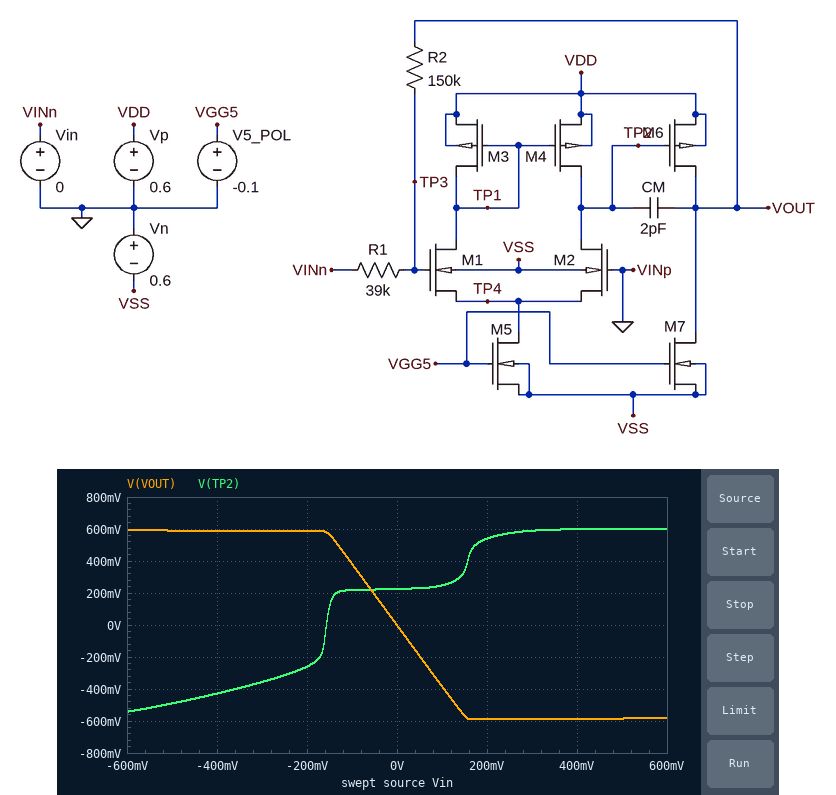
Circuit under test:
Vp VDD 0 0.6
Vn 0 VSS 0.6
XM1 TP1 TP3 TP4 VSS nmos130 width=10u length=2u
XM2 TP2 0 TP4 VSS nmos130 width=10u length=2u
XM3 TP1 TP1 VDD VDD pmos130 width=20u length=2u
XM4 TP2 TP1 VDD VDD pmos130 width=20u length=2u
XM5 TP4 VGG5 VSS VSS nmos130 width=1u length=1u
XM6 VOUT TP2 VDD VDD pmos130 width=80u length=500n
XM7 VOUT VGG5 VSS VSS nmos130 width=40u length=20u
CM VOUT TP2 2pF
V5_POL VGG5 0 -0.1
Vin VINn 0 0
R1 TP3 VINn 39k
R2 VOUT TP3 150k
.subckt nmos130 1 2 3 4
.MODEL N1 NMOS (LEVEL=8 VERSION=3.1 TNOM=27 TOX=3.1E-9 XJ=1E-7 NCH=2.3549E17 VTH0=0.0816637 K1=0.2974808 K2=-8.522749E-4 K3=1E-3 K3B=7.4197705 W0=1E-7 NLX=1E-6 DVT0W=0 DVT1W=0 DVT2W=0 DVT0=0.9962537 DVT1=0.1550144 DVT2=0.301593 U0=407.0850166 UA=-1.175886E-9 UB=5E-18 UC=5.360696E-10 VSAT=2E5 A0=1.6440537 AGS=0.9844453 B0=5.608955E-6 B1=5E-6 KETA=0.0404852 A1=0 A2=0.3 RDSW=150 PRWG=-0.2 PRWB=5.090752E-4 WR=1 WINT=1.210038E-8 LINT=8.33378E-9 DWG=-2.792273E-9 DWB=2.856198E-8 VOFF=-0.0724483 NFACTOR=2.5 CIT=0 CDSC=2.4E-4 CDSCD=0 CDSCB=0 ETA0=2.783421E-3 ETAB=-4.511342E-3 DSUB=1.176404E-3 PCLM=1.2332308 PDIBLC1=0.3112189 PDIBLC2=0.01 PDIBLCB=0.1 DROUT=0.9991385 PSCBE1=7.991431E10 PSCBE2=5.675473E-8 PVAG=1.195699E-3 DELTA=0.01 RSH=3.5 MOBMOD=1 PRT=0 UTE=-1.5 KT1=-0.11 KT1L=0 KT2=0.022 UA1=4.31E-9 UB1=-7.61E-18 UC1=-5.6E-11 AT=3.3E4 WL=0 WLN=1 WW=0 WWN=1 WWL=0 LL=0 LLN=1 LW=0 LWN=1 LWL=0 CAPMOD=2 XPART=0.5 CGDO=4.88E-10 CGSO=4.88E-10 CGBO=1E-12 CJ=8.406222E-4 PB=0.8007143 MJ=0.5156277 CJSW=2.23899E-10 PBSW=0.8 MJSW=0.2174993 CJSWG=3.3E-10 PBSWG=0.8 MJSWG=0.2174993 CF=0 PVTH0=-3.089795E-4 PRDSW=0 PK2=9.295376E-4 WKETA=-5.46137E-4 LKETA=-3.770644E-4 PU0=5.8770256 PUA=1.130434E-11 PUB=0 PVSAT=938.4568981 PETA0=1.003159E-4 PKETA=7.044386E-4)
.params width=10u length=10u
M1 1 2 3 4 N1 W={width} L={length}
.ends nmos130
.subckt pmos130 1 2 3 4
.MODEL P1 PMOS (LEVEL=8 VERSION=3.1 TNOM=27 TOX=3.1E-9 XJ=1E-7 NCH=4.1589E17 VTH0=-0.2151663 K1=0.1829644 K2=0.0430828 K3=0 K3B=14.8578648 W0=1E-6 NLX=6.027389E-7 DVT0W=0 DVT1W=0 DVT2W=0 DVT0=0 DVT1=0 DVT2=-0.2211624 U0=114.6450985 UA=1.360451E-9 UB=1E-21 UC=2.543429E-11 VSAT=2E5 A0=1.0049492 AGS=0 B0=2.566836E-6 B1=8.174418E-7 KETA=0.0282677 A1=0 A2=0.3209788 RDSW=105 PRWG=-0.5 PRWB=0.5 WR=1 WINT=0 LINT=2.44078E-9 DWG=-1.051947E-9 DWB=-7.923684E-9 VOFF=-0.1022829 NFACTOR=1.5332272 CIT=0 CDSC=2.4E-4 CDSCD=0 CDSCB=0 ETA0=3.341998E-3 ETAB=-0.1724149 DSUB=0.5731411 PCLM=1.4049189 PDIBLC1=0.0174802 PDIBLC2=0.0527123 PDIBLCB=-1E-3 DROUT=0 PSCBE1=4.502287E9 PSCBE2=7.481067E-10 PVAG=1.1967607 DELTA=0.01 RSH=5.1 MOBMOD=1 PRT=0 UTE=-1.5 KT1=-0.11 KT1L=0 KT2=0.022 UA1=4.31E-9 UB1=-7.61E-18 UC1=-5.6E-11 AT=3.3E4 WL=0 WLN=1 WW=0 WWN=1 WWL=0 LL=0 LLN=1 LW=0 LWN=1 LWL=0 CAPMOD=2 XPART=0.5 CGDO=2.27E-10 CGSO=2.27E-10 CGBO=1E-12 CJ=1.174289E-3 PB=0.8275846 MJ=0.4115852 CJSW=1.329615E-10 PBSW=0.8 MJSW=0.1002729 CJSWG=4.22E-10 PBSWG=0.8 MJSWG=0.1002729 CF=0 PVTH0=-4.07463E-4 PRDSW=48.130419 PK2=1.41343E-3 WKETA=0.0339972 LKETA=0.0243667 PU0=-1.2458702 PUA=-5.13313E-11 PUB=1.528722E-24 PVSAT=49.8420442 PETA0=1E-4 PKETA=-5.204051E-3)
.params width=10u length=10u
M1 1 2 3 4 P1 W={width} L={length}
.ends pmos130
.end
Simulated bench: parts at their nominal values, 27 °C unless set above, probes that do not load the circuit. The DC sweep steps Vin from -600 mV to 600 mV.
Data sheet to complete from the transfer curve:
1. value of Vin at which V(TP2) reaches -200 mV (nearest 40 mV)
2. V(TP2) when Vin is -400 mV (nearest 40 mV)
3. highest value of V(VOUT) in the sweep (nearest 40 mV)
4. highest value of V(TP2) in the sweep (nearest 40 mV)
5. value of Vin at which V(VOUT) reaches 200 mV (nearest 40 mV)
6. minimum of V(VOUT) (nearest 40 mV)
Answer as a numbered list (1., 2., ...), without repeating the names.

1. -160 mV
2. -440 mV
3. 600 mV
4. 600 mV
5. -40 mV
6. -600 mV
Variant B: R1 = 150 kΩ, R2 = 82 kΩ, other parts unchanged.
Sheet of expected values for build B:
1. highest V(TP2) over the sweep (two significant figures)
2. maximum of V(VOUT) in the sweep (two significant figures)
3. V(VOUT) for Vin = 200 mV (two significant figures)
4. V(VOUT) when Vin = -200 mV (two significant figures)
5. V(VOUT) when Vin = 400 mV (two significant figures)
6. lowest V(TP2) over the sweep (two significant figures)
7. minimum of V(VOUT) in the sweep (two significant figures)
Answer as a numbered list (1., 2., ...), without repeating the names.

1. 240 mV
2. 330 mV
3. -110 mV
4. 110 mV
5. -220 mV
6. 220 mV
7. -330 mV
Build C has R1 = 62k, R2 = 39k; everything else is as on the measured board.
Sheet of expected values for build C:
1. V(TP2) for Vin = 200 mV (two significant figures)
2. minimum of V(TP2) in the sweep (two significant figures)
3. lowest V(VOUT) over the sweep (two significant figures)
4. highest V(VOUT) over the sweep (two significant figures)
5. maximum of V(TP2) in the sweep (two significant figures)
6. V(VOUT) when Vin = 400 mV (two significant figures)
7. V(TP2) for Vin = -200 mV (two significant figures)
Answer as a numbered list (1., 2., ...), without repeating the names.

1. 230 mV
2. 210 mV
3. -380 mV
4. 380 mV
5. 250 mV
6. -250 mV
7. 220 mV
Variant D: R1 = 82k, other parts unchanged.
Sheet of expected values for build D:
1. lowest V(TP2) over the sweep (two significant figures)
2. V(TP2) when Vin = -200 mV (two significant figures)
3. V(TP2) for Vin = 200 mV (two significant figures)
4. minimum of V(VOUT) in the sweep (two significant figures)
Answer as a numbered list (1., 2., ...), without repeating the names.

1. -410 mV
2. 220 mV
3. 240 mV
4. -590 mV
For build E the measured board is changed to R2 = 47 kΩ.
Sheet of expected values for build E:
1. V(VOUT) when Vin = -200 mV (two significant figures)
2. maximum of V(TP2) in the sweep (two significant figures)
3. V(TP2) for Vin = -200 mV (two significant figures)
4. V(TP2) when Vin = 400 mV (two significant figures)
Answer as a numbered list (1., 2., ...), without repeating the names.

1. 240 mV
2. 570 mV
3. 220 mV
4. 280 mV
